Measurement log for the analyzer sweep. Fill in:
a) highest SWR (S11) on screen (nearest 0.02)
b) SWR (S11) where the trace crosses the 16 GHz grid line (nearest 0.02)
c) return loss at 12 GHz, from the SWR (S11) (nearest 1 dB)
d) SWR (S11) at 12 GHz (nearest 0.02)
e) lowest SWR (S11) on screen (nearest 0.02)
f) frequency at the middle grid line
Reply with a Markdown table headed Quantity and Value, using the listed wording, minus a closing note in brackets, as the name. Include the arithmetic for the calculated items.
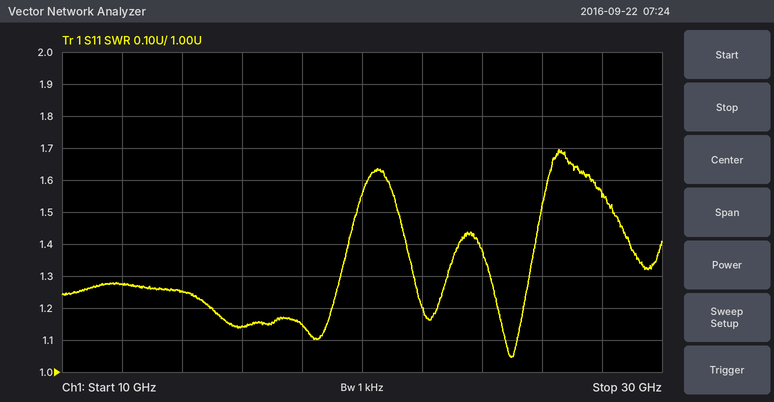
| Quantity | Value |
|---|---|
| highest SWR (S11) on screen | 1.70 |
| SWR (S11) where the trace crosses the 16 GHz grid line | 1.14 |
| return loss at 12 GHz, from the SWR (S11) | −20 log10((1.28 − 1)/(1.28 + 1)) ≈ 18 dB |
| SWR (S11) at 12 GHz | 1.28 |
| lowest SWR (S11) on screen | 1.04 |
| frequency at the middle grid line | 20 GHz |
